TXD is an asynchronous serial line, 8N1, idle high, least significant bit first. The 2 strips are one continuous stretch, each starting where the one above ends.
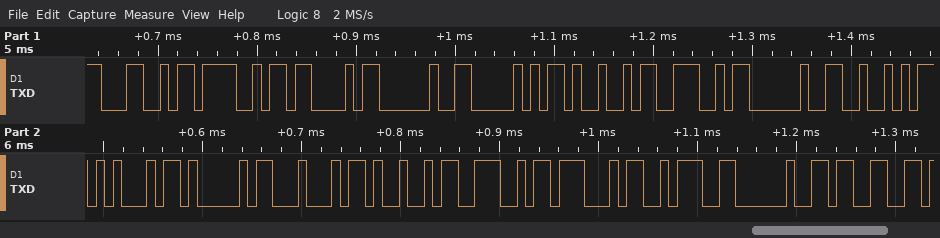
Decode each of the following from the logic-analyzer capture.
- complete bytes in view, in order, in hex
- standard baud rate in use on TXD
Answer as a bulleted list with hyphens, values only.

- 0x4C 0x4F 0x43 0x20 0x50 0x49 0x4E 0x20 0x52 0x45 0x41 0x44 0x49 0x4E 0x47 0x3A 0x20 0x33
- 115200 baud
